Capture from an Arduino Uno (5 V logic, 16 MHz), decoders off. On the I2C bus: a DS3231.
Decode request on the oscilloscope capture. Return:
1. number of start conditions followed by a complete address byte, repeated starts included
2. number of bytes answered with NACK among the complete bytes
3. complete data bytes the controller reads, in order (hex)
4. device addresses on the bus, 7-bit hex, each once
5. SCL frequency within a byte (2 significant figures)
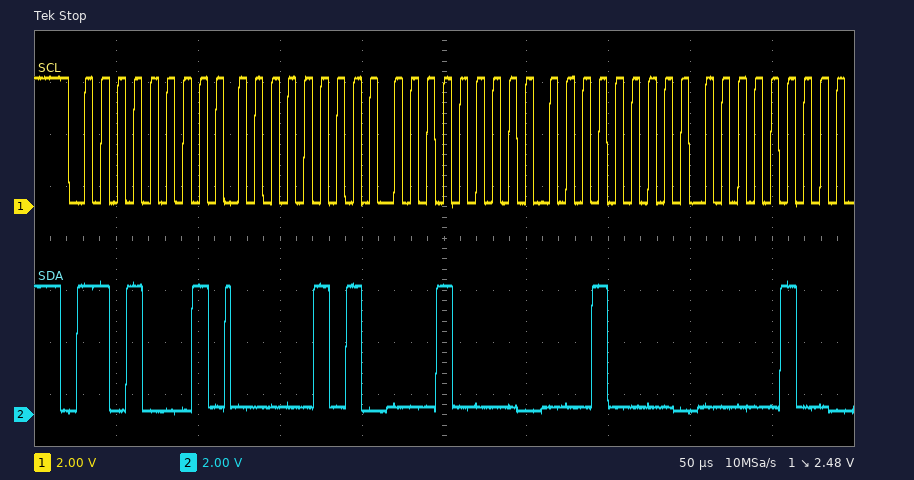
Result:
1
0
05 10 10 04
0x68
100 kHz
